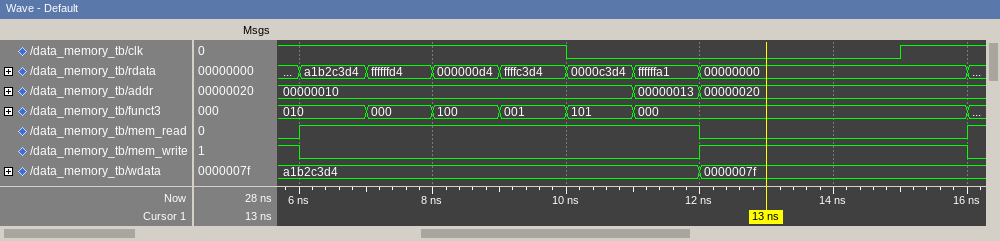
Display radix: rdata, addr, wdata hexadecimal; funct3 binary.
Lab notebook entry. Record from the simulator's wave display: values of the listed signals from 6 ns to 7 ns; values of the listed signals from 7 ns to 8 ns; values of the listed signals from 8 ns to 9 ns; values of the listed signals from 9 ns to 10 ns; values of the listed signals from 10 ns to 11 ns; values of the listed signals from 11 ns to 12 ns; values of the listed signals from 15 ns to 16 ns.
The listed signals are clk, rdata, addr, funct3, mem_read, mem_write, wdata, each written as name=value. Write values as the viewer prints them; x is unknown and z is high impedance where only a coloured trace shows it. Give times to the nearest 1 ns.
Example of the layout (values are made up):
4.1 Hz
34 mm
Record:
clk=1, rdata=a1b2c3d4, addr=00000010, funct3=010, mem_read=1, mem_write=0, wdata=a1b2c3d4
clk=1, rdata=ffffffd4, addr=00000010, funct3=000, mem_read=1, mem_write=0, wdata=a1b2c3d4
clk=1, rdata=000000d4, addr=00000010, funct3=100, mem_read=1, mem_write=0, wdata=a1b2c3d4
clk=1, rdata=ffffc3d4, addr=00000010, funct3=001, mem_read=1, mem_write=0, wdata=a1b2c3d4
clk=0, rdata=0000c3d4, addr=00000010, funct3=101, mem_read=1, mem_write=0, wdata=a1b2c3d4
clk=0, rdata=ffffffa1, addr=00000013, funct3=000, mem_read=1, mem_write=0, wdata=a1b2c3d4
clk=1, rdata=00000000, addr=00000020, funct3=000, mem_read=0, mem_write=1, wdata=0000007f
